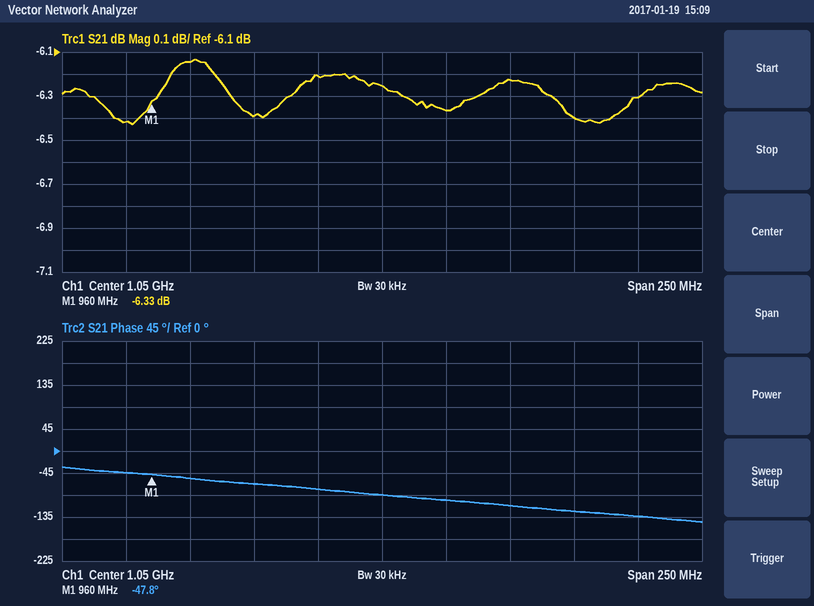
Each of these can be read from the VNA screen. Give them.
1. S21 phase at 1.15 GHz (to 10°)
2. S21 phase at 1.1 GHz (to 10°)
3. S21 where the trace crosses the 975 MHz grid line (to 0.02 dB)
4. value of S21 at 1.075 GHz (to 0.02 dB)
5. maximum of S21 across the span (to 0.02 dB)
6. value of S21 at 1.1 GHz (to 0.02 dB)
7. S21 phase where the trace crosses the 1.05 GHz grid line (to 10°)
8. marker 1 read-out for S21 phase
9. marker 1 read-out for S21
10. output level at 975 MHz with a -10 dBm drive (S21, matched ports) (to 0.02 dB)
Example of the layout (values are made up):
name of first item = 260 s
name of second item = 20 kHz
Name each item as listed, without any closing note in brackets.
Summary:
S21 phase at 1.15 GHz = -130°
S21 phase at 1.1 GHz = -110°
S21 where the trace crosses the 975 MHz grid line = -6.14 dB
value of S21 at 1.075 GHz = -6.36 dB
maximum of S21 across the span = -6.14 dB
value of S21 at 1.1 GHz = -6.22 dB
S21 phase where the trace crosses the 1.05 GHz grid line = -90°
marker 1 read-out for S21 phase = -47.8°
marker 1 read-out for S21 = -6.33 dB
output level at 975 MHz with a -10 dBm drive (S21, matched ports) = -16.14 dBm
